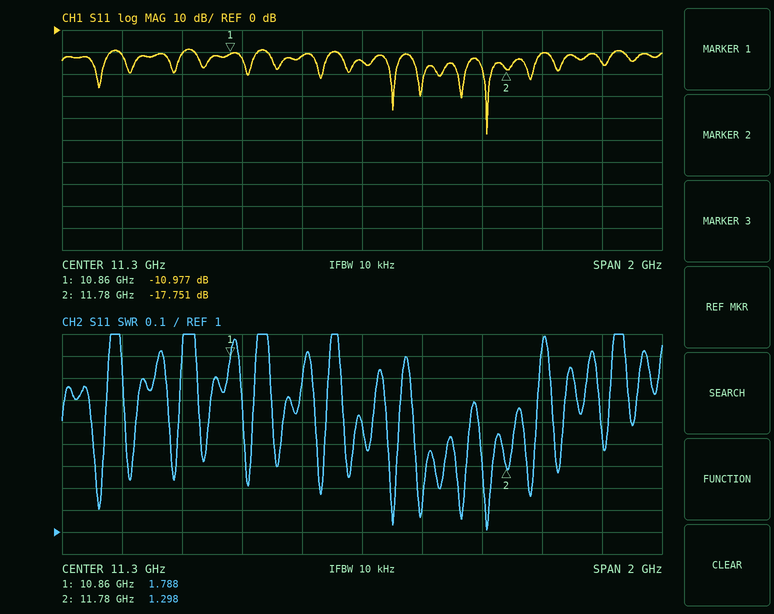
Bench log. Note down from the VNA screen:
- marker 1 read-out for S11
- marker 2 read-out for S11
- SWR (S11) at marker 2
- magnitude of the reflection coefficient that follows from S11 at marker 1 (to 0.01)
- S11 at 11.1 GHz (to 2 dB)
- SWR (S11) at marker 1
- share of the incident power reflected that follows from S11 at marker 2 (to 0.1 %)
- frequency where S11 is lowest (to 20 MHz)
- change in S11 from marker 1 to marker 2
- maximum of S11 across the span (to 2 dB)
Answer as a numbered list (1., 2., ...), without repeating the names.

1. -10.977 dB
2. -17.751 dB
3. 1.298
4. 0.28
5. -12 dB
6. 1.788
7. 1.7 %
8. 11.72 GHz
9. -6.774 dB
10. -8 dB
